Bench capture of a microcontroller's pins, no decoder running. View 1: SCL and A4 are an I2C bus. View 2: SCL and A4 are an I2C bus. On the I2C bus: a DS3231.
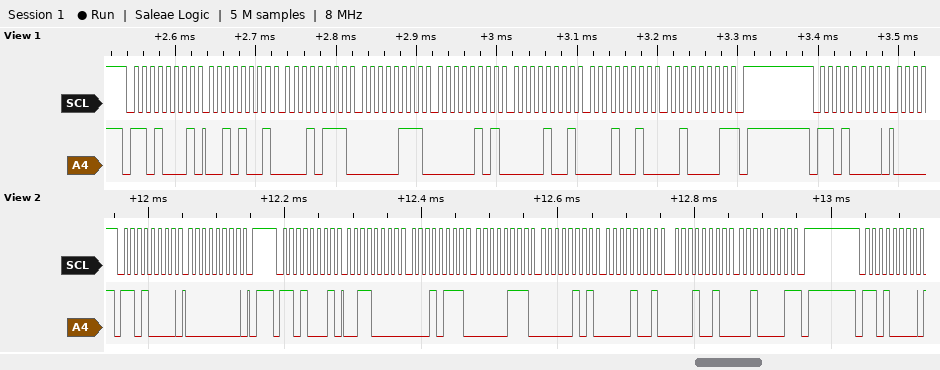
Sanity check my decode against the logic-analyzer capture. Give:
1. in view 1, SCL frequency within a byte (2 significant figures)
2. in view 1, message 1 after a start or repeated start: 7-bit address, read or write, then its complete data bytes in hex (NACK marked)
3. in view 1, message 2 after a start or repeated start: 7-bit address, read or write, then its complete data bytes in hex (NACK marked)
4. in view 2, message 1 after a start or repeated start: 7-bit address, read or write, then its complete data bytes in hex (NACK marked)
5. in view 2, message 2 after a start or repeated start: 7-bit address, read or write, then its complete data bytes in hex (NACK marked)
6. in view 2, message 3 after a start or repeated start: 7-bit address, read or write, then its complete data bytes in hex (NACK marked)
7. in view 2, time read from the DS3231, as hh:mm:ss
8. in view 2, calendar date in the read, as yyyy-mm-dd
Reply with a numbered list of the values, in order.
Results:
1. 100 kHz
2. 0x68 read: 29 17 07 05 09 12 21 NACK
3. 0x68 write
4. 0x68 write: 00
5. 0x68 read: 30 17 07 05 09 12 21 NACK
6. 0x68 write
7. 07:17:30
8. 2021-12-09
